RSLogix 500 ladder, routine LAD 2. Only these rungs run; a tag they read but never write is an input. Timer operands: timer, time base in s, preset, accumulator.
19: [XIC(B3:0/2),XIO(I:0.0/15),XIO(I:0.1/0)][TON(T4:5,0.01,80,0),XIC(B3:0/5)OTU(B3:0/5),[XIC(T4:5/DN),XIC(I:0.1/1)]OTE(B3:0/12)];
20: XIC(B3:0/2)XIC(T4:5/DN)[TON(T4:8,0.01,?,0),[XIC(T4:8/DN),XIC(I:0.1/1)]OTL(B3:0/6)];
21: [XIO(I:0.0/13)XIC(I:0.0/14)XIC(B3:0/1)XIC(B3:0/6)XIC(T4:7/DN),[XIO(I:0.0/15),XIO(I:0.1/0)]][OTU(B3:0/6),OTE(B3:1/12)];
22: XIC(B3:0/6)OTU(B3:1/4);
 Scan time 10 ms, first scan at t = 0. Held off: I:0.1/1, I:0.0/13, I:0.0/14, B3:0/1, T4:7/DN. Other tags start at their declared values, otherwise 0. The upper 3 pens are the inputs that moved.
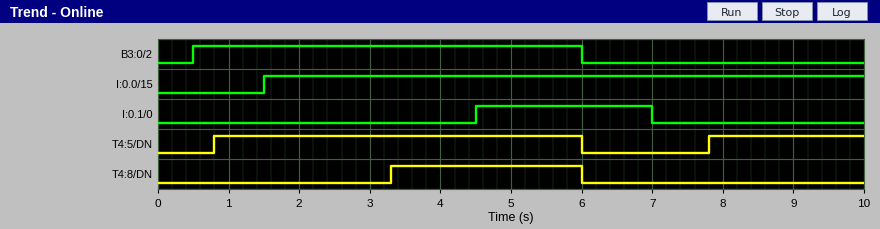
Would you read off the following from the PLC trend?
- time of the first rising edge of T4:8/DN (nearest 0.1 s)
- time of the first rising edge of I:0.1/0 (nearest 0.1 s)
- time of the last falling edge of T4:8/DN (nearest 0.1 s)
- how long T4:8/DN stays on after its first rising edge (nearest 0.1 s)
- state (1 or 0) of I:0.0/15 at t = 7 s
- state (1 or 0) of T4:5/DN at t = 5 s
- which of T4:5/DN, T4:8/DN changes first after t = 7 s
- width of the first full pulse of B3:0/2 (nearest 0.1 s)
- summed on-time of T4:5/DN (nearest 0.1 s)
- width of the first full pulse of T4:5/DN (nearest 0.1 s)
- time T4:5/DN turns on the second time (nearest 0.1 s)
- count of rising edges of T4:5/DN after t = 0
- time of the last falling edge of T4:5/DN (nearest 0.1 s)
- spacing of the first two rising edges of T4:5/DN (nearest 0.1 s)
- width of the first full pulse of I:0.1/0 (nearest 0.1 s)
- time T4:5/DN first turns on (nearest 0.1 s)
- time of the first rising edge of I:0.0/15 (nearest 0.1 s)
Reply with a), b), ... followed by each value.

a) 3.3 s
b) 4.5 s
c) 6.0 s
d) 2.7 s
e) 1
f) 1
g) T4:5/DN
h) 5.5 s
i) 7.4 s
j) 5.2 s
k) 7.8 s
l) 2
m) 6.0 s
n) 7.0 s
o) 2.5 s
p) 0.8 s
q) 1.5 s
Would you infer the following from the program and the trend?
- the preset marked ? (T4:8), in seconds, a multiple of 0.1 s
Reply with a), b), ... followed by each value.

a) 2.5 s
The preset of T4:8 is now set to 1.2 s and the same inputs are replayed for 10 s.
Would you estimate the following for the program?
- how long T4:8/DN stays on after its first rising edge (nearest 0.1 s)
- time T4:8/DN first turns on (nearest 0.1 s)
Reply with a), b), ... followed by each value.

a) 4.0 s
b) 2.0 s
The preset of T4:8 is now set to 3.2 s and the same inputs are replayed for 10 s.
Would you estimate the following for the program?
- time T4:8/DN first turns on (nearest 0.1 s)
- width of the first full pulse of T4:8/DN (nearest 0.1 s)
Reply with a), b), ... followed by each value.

a) 4.0 s
b) 2.0 s
